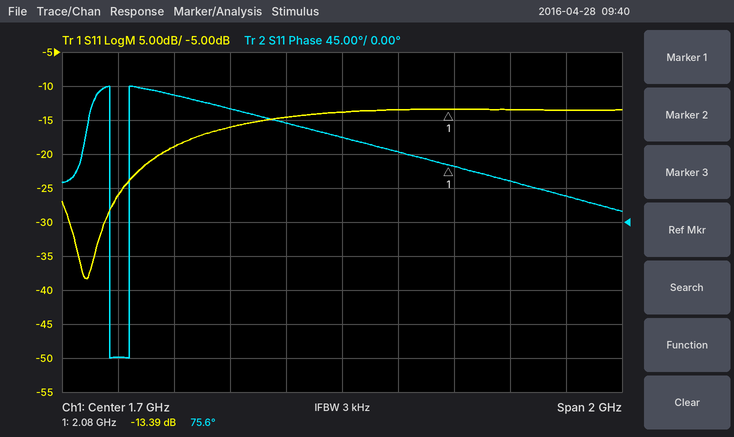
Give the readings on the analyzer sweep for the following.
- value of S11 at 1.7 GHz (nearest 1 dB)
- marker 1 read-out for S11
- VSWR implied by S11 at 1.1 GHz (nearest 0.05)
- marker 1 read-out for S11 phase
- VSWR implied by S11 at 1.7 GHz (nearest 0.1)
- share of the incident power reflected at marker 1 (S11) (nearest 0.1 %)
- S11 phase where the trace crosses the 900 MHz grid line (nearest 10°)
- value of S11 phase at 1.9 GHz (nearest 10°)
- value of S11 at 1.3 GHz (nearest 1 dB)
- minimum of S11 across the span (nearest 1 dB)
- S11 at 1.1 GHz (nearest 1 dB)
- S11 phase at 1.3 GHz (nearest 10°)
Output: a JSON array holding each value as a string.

["-14 dB", "-13.39 dB", "1.25", "75.6°", "1.5", "4.6 %", "-180°", "90°", "-16 dB", "-38 dB", "-19 dB", "150°"]
